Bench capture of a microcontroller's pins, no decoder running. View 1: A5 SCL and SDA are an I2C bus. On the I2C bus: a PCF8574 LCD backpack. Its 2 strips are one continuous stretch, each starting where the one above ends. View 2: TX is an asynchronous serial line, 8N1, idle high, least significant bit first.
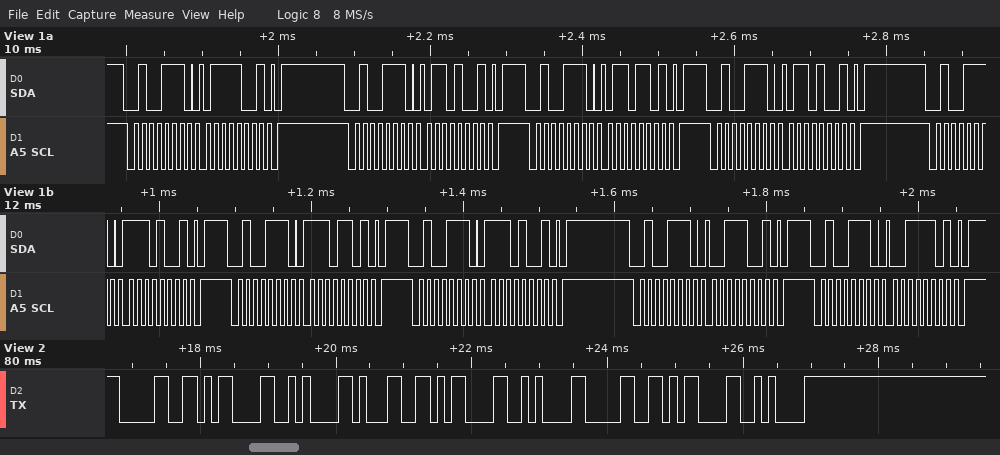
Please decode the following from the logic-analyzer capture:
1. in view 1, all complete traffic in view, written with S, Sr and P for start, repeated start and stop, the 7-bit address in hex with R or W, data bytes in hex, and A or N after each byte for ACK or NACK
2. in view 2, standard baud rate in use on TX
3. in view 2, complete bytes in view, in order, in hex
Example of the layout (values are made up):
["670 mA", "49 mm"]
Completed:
["S 27W A 79 A P S 27W A 69 A P S 27W A 6D A P S 27W A 69 A P S 27W A E9 A P S 27W A ED A P S 27W A E9 A P S 27W A 39 A P S 27W A 3D A P", "9600 baud", "30 0D 0A 31 0D 0A 30 0D 0A"]
